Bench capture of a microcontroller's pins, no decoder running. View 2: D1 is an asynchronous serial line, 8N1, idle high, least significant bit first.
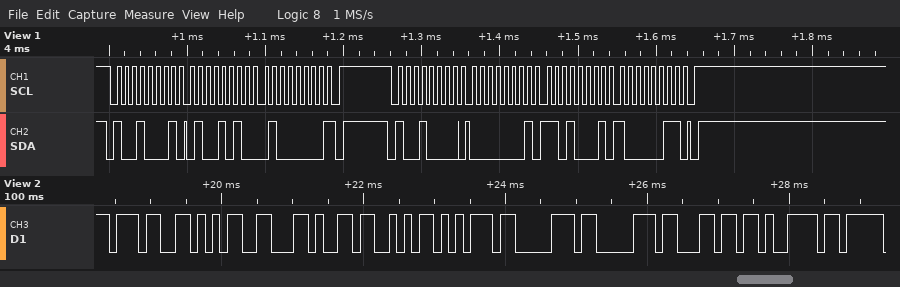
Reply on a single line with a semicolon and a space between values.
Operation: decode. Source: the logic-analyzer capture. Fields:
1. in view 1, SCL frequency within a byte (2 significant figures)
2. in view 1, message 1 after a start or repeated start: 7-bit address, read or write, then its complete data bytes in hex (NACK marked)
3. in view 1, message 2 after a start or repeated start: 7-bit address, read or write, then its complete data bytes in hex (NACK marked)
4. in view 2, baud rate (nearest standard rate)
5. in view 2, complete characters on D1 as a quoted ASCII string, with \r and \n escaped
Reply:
100 kHz; 0x48 read: 4A 40 NACK; 0x48 write: 01 D1 83; 9600 baud; "75,Supply"
